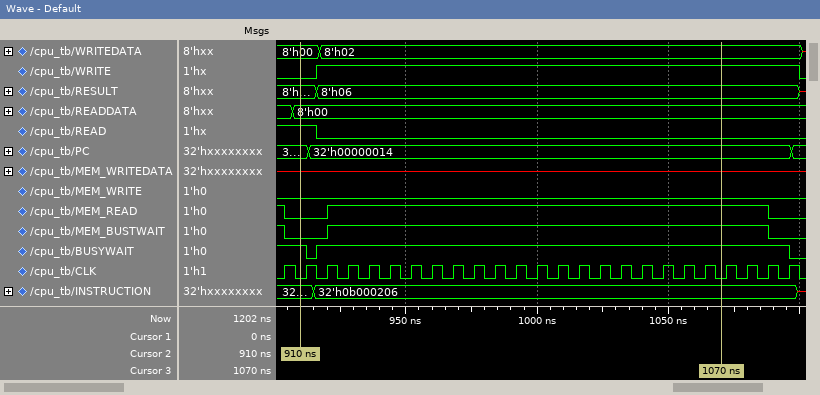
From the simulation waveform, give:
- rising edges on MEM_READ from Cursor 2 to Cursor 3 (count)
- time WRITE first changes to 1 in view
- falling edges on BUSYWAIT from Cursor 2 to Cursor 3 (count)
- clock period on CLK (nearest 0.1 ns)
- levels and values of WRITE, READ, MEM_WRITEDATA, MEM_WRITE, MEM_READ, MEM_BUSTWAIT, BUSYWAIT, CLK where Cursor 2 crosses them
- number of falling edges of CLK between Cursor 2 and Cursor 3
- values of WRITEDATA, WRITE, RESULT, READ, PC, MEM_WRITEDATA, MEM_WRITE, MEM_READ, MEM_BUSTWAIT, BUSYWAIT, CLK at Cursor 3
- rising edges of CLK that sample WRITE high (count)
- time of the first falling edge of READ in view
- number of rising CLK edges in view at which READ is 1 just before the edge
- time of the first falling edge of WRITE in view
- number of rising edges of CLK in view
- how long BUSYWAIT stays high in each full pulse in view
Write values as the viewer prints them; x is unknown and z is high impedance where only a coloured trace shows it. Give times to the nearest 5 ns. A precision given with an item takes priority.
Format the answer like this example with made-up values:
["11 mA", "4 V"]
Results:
["1", "915 ns", "1", "8 ns", "WRITE=0, READ=1, MEM_WRITEDATA=x, MEM_WRITE=0, MEM_READ=0, MEM_BUSTWAIT=0, BUSYWAIT=1, CLK=0", "20", "WRITEDATA=8'h02, WRITE=1, RESULT=8'h06, READ=0, PC=32'h00000014, MEM_WRITEDATA=x, MEM_WRITE=0, MEM_READ=1, MEM_BUSTWAIT=1, BUSYWAIT=1, CLK=0", "23", "915 ns", "2", "1100 ns", "25", "180 ns"]
